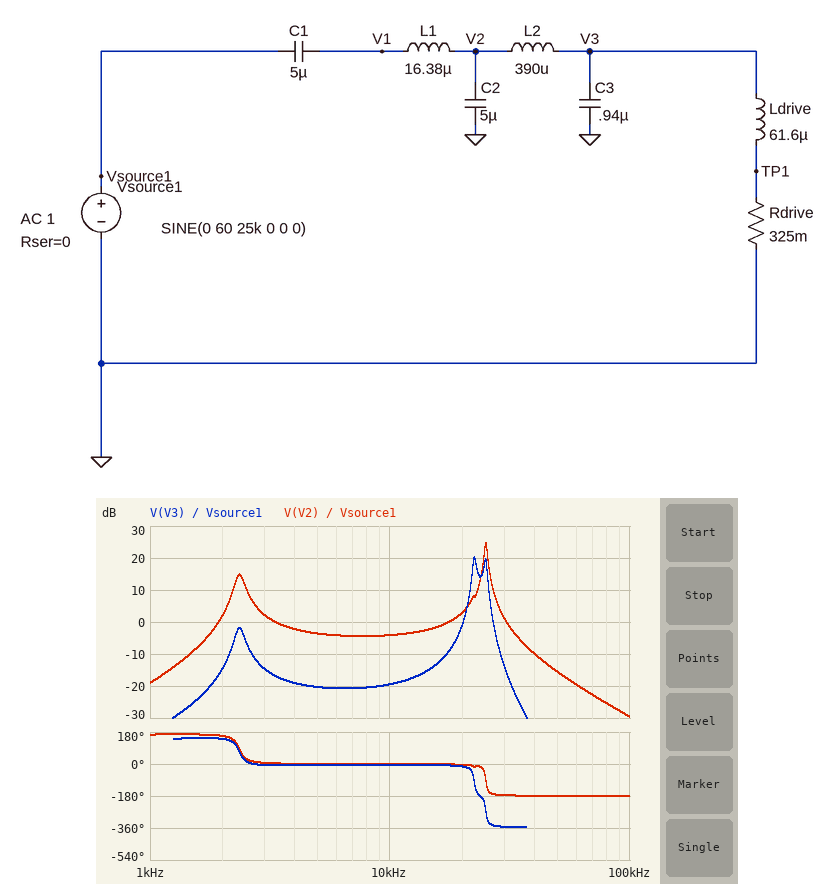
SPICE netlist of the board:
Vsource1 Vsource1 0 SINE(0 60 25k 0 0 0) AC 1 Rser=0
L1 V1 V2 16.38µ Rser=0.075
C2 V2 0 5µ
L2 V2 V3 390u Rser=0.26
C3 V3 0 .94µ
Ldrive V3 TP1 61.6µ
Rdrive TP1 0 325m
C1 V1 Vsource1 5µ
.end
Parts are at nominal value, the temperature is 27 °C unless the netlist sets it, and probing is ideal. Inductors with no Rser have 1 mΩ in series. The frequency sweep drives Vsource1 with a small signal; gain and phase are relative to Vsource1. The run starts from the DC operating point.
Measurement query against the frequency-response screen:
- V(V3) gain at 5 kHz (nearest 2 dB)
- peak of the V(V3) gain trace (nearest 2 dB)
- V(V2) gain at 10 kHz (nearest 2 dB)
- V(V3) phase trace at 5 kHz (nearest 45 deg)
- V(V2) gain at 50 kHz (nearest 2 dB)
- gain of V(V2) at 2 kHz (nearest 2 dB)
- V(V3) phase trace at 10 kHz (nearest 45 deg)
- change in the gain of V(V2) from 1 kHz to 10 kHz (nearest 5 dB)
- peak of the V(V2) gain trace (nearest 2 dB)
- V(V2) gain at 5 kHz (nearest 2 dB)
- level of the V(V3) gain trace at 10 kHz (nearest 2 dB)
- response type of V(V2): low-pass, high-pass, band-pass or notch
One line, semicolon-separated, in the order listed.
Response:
-20 dB; 20 dB; -4 dB; 0 deg; -16 dB; 2 dB; 0 deg; 15 dB; 24 dB; -4 dB; -20 dB; band-pass
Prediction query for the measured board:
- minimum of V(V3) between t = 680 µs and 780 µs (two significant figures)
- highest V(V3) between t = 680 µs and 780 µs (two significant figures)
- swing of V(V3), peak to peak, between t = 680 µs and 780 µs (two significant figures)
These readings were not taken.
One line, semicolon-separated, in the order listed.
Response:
-480 V; 480 V; 960 V
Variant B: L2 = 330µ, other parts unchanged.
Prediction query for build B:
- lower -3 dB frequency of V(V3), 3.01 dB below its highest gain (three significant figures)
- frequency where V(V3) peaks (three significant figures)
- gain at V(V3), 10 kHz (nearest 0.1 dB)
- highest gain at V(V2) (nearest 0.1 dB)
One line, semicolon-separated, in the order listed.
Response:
22.4 kHz; 22.7 kHz; -18.2 dB; 24.5 dB
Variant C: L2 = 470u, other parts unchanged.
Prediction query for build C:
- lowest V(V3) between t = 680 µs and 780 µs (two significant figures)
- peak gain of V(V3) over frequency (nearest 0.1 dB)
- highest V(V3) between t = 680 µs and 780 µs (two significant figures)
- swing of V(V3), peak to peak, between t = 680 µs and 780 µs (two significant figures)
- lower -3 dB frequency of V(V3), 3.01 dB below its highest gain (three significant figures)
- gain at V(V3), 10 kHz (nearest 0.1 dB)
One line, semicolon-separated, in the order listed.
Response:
-360 V; 18.0 dB; 360 V; 720 V; 21.9 kHz; -20.9 dB
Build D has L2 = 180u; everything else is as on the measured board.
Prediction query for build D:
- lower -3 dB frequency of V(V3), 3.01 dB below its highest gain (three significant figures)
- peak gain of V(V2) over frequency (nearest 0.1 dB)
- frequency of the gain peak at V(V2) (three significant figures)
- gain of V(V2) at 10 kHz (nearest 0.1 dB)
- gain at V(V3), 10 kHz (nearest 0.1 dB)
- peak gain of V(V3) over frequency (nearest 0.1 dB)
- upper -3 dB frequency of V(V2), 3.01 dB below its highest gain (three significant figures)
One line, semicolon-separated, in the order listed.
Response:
23.4 kHz; 22.6 dB; 25.8 kHz; -3.8 dB; -14.0 dB; 28.5 dB; 26.1 kHz
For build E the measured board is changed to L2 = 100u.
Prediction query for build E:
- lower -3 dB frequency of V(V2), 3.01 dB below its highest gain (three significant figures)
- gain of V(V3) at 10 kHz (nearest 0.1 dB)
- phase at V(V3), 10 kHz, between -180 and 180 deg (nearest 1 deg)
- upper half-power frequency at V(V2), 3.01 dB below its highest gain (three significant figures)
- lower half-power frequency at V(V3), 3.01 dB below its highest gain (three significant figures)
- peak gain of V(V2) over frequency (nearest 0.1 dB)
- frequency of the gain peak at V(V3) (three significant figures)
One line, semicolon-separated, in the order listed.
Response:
23.8 kHz; -10.5 dB; -2 deg; 24.6 kHz; 23.9 kHz; 21.2 dB; 24.3 kHz
